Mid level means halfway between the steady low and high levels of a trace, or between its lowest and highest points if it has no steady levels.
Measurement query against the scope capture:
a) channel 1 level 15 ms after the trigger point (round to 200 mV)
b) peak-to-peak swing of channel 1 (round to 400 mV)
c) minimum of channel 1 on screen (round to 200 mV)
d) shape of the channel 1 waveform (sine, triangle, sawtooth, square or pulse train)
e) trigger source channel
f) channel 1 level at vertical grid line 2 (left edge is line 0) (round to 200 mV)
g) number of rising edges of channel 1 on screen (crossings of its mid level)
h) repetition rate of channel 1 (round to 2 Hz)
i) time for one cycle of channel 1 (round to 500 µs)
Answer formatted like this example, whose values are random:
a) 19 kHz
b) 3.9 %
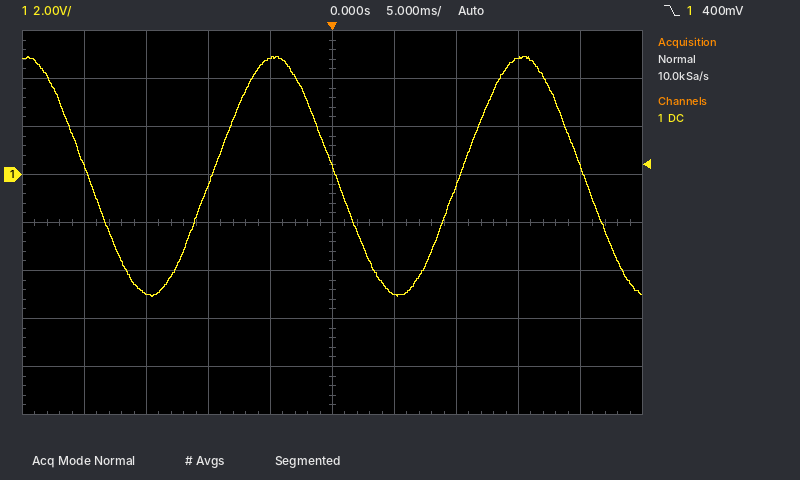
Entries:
a) 4.8 V
b) 10.0 V
c) -5.0 V
d) sine
e) channel 1
f) -5.0 V
g) 2
h) 50 Hz
i) 20.0 ms
